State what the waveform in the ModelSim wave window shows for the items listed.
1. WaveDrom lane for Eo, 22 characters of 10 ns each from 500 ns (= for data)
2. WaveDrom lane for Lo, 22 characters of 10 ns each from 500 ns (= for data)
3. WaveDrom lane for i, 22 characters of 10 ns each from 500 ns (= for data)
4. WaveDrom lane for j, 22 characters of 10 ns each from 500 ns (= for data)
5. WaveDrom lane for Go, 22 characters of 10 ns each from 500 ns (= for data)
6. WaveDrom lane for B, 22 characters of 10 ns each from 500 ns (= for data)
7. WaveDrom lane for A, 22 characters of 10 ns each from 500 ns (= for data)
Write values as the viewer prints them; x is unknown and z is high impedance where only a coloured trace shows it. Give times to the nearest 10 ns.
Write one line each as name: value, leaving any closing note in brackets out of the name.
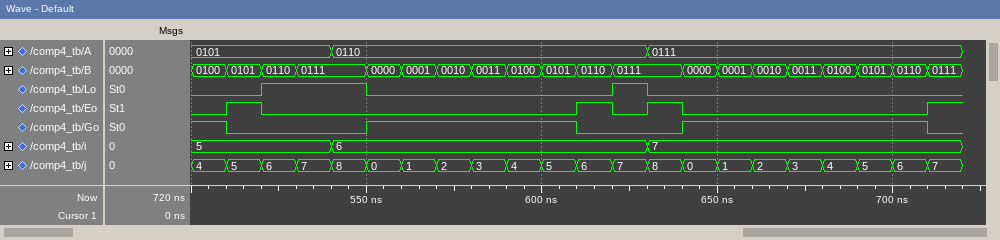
WaveDrom lane for Eo, 22 characters of 10 ns each from 500 ns: {name: 'Eo', wave: '010........1010......1'}
WaveDrom lane for Lo, 22 characters of 10 ns each from 500 ns: {name: 'Lo', wave: '0.1..0......10........'}
WaveDrom lane for i, 22 characters of 10 ns each from 500 ns: {name: 'i', wave: '=...=........=........', data: '5 6 7'}
WaveDrom lane for j, 22 characters of 10 ns each from 500 ns: {name: 'j', wave: '======================', data: '4 5 6 7 8 0 1 2 3 4 5 6 7 8 0 1 2 3 4 5 6 7'}
WaveDrom lane for Go, 22 characters of 10 ns each from 500 ns: {name: 'Go', wave: '10...1.....0..1......0'}
WaveDrom lane for B, 22 characters of 10 ns each from 500 ns: {name: 'B', wave: '====.========.========', data: '0100 0101 0110 0111 0000 0001 0010 0011 0100 0101 0110 0111 0000 0001 0010 0011 0100 0101 0110 0111'}
WaveDrom lane for A, 22 characters of 10 ns each from 500 ns: {name: 'A', wave: '=...=........=........', data: '0101 0110 0111'}
